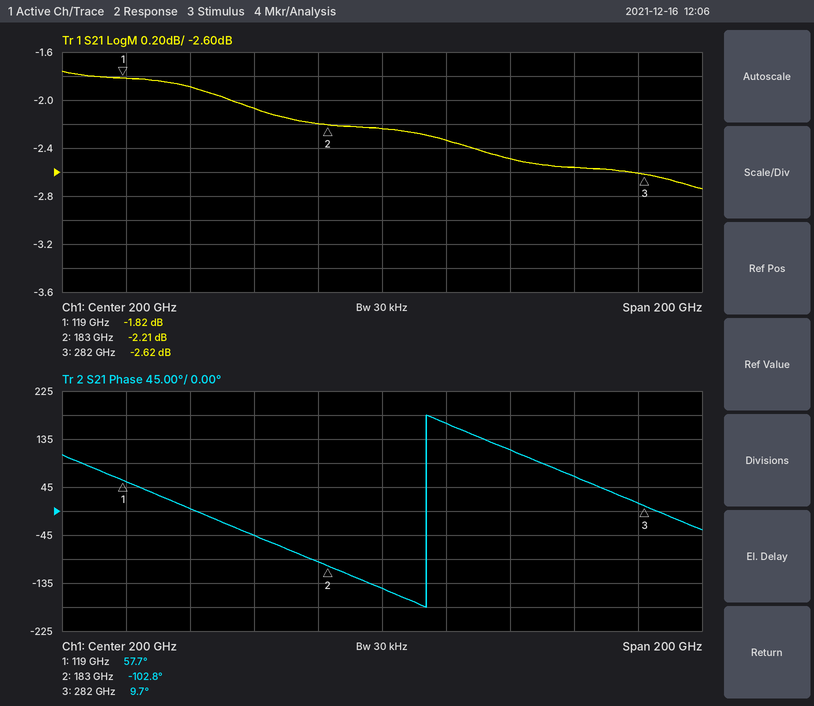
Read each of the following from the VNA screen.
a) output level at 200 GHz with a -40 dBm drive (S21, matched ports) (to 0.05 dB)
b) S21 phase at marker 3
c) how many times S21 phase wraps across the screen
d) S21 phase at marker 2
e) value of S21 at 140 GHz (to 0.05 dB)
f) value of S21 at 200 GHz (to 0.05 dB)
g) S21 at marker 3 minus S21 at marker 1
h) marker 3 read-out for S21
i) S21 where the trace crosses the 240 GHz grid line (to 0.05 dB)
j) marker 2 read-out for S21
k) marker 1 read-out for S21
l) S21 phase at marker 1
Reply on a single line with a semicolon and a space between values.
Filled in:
-42.25 dBm; 9.7°; 1; -102.8°; -1.90 dB; -2.25 dB; -0.80 dB; -2.62 dB; -2.50 dB; -2.21 dB; -1.82 dB; 57.7°
